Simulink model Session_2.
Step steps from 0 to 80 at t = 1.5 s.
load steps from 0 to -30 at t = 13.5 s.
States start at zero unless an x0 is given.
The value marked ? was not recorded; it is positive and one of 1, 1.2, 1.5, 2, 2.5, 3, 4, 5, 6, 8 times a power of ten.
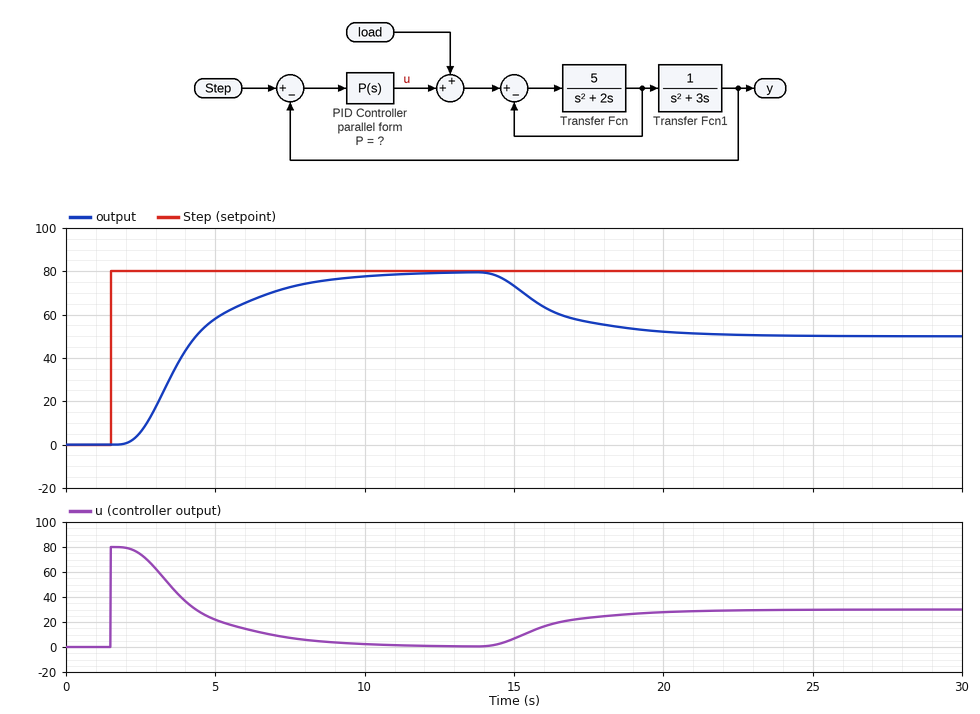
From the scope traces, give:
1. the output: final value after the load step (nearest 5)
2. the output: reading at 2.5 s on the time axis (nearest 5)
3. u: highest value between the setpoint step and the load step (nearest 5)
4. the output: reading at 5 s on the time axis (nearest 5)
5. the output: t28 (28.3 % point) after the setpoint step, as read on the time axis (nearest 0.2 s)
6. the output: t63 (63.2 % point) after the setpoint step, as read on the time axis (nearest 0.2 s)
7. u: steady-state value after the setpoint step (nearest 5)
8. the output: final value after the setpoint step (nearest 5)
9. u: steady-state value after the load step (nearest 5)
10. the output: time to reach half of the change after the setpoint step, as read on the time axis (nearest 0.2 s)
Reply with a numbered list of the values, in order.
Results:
1. 50
2. 5
3. 80
4. 60
5. 3.2 s
6. 4.4 s
7. 0
8. 80
9. 30
10. 3.8 s
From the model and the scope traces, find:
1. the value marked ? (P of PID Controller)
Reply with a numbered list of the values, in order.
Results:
1. 1
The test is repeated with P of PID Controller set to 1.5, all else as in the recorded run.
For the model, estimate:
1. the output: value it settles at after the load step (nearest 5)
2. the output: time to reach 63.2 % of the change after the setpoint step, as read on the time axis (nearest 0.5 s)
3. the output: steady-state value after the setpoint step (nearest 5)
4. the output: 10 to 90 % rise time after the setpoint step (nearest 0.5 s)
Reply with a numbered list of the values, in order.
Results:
1. 60
2. 3.5 s
3. 80
4. 2.0 s
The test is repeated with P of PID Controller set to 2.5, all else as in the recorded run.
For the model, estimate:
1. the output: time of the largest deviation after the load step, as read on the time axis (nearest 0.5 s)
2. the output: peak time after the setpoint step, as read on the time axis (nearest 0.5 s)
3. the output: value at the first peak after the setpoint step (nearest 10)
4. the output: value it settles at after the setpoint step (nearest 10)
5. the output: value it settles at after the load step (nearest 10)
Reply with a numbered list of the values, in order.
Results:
1. 16.5 s
2. 4.5 s
3. 100
4. 80
5. 70
